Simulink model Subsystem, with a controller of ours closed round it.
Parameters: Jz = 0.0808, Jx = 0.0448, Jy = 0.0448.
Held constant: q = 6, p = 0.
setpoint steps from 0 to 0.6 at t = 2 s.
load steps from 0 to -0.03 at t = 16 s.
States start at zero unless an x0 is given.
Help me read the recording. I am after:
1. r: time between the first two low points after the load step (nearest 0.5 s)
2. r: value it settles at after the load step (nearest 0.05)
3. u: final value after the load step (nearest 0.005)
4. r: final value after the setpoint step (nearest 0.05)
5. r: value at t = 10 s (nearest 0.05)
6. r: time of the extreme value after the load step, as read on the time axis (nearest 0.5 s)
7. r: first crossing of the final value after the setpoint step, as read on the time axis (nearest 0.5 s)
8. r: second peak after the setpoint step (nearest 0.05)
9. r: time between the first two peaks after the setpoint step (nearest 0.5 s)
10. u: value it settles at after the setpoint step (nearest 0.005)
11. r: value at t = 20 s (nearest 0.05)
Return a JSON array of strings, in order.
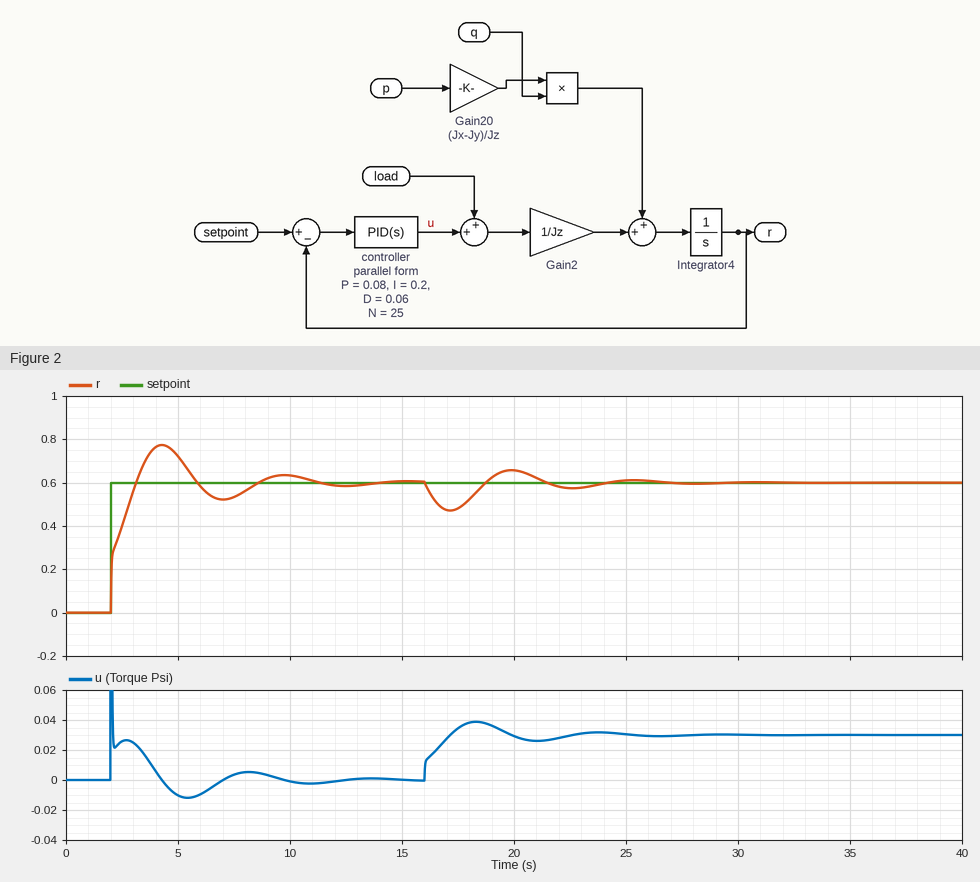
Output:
["5.5 s", "0.60", "0.030", "0.60", "0.65", "17.0 s", "3.0 s", "0.65", "5.5 s", "0.000", "0.65"]
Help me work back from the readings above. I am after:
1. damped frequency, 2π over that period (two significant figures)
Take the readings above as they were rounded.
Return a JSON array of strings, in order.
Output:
["1.1 rad/s"]
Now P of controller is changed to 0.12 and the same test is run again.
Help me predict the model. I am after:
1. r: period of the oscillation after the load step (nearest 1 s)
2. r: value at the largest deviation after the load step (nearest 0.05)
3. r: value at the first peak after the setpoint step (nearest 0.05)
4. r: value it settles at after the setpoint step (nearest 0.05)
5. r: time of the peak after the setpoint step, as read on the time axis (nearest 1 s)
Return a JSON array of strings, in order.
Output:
["6 s", "0.50", "0.75", "0.60", "4 s"]
